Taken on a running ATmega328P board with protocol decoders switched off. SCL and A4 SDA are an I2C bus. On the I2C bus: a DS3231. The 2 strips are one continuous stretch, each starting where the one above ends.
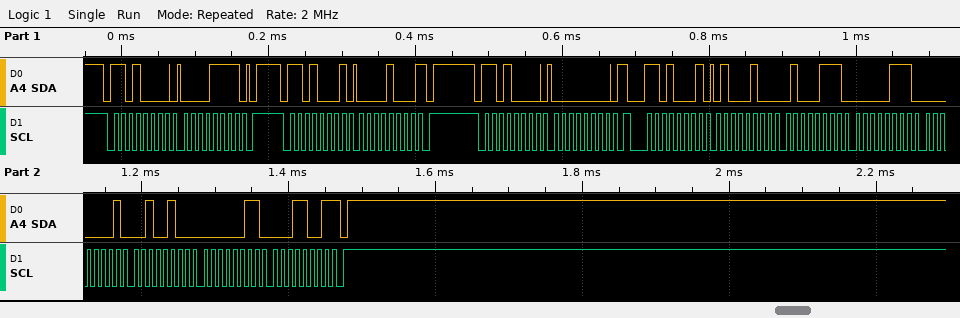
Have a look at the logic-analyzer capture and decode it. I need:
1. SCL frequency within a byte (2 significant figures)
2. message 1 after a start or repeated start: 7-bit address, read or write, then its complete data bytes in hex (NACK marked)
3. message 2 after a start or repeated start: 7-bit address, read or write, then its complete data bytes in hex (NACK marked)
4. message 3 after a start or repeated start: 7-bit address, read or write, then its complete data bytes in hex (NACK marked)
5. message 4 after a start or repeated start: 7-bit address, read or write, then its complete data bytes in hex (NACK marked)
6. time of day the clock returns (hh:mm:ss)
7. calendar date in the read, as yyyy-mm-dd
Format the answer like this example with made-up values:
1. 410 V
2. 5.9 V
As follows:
1. 100 kHz
2. 0x68 write: 0F
3. 0x68 read: 08 NACK
4. 0x68 write: 00
5. 0x68 read: 44 47 07 01 24 03 19 NACK
6. 07:47:44
7. 2019-03-24
